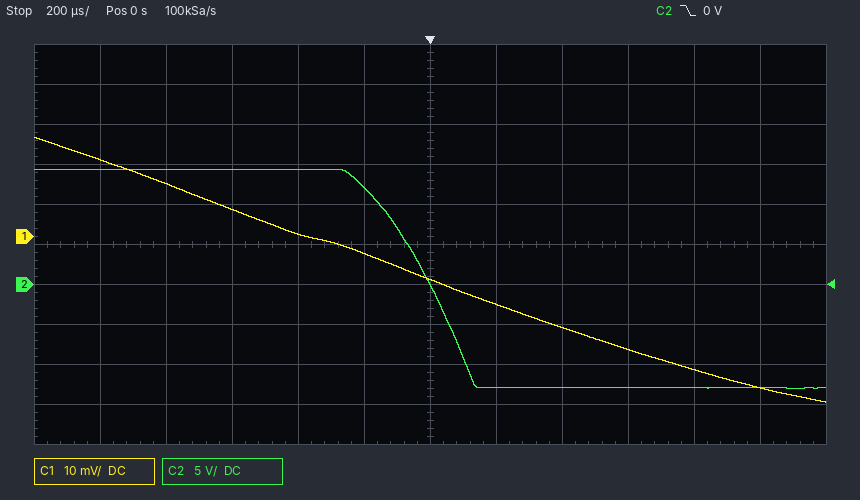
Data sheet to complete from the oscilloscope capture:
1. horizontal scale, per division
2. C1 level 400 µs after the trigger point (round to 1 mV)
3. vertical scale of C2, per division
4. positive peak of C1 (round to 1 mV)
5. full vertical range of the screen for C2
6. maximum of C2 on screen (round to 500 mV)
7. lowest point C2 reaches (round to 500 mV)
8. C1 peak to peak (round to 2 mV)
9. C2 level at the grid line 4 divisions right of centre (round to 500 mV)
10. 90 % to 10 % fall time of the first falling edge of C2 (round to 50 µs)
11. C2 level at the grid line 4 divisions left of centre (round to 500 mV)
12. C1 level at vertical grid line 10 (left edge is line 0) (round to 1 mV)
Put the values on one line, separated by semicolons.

200 µs; -23 mV; 5 V; 25 mV; 50 V; 14.5 V; -13.0 V; 66 mV; -13.0 V; 300 µs; 14.5 V; -33 mV
